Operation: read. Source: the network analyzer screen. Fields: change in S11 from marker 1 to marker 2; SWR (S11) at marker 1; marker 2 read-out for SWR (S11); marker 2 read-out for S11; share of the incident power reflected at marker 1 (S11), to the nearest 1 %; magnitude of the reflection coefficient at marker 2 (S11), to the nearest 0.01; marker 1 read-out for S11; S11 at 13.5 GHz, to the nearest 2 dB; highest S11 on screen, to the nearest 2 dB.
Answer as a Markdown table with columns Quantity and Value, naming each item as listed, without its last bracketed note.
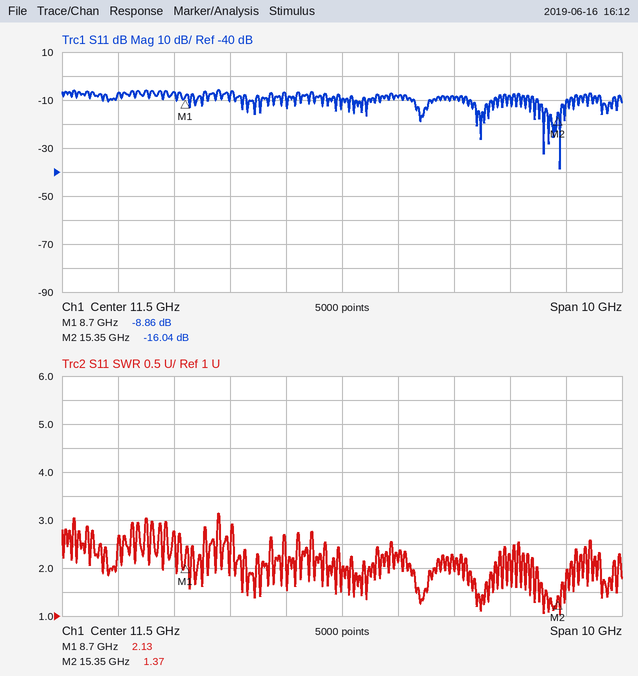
| Quantity | Value |
|---|---|
| change in S11 from marker 1 to marker 2 | -7.18 dB |
| SWR (S11) at marker 1 | 2.13 |
| marker 2 read-out for SWR | 1.37 |
| marker 2 read-out for S11 | -16.04 dB |
| share of the incident power reflected at marker 1 (S11), to the nearest 1 % | 13 % |
| magnitude of the reflection coefficient at marker 2 (S11), to the nearest 0.01 | 0.16 |
| marker 1 read-out for S11 | -8.86 dB |
| S11 at 13.5 GHz, to the nearest 2 dB | -10 dB |
| highest S11 on screen, to the nearest 2 dB | -6 dB |
